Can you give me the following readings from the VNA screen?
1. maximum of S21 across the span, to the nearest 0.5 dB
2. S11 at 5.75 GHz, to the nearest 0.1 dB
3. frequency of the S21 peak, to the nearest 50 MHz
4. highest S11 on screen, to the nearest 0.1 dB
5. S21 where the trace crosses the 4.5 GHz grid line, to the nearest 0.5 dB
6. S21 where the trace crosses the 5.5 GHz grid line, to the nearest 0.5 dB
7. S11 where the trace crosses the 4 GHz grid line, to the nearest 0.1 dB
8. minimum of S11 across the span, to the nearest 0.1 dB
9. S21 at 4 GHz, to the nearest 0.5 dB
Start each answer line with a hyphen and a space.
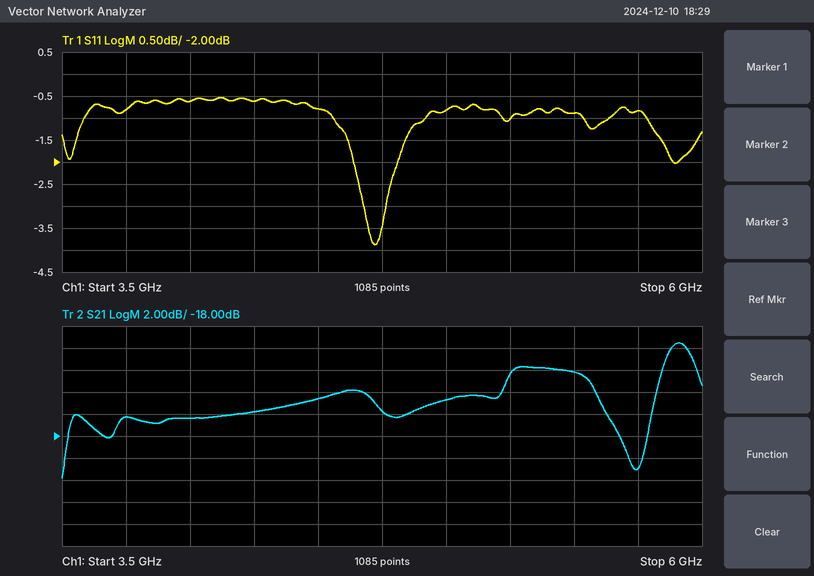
- -9.5 dB
- -0.8 dB
- 5.90 GHz
- -0.5 dB
- -14.5 dB
- -12.0 dB
- -0.6 dB
- -3.9 dB
- -16.5 dB
